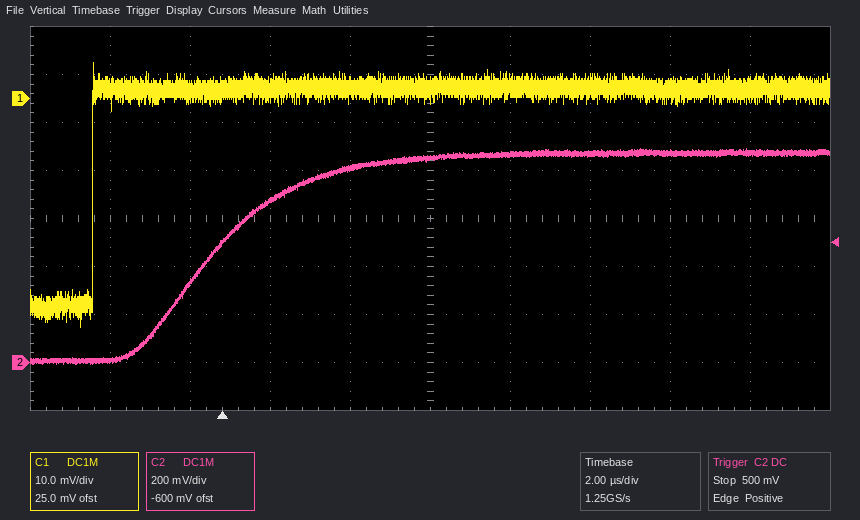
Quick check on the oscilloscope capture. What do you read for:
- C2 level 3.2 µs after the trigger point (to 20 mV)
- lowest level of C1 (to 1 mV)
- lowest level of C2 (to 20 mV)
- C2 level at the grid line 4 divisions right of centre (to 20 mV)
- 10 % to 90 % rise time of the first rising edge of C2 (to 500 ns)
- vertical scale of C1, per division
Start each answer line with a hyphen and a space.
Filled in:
- 800 mV
- -48 mV
- 0 mV
- 880 mV
- 4.5 µs
- 10 mV
